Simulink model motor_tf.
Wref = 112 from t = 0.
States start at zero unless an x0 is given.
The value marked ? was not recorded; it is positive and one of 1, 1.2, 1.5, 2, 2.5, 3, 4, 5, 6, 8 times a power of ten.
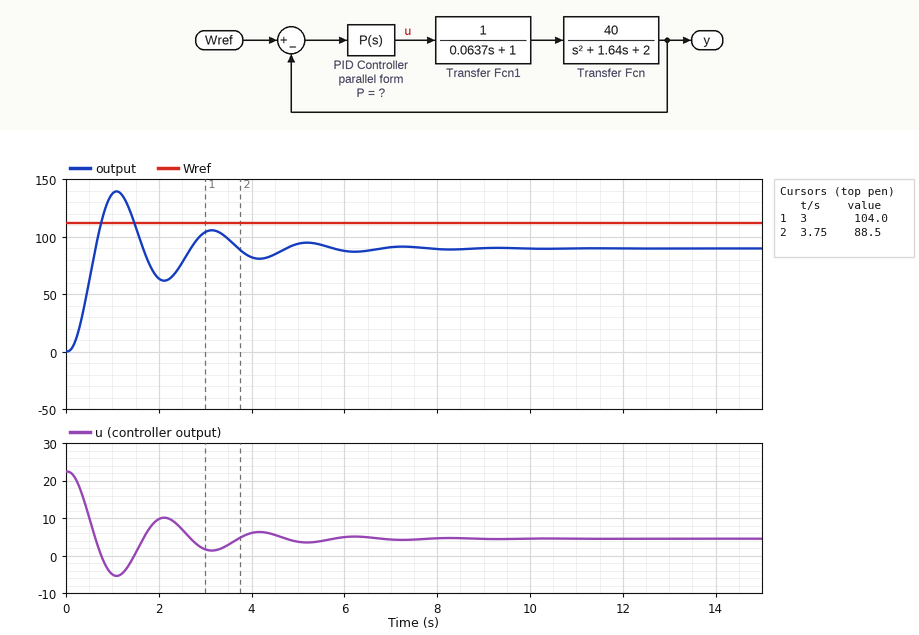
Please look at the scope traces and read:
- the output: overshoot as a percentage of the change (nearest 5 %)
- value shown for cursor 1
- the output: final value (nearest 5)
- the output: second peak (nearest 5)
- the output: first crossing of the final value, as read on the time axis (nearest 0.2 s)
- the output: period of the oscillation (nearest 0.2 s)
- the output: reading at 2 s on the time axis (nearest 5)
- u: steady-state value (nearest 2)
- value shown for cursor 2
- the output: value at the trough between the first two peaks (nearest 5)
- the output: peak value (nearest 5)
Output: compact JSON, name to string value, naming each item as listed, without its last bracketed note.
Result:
{"the output: overshoot as a percentage of the change": "55 %", "value shown for cursor 1": "104.0", "the output: final value": "90", "the output: second peak": "105", "the output: first crossing of the final value, as read on the time axis": "0.6 s", "the output: period of the oscillation": "2.0 s", "the output: reading at 2 s on the time axis": "65", "u: steady-state value": "4", "value shown for cursor 2": "88.5", "the output: value at the trough between the first two peaks": "60", "the output: peak value": "140"}
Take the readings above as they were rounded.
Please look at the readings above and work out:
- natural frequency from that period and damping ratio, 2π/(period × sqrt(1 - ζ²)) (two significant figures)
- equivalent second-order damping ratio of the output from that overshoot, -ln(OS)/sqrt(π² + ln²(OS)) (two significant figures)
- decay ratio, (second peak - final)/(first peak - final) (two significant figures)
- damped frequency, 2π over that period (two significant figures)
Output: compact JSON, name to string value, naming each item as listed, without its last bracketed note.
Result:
{"natural frequency from that period and damping ratio, 2π/(period × sqrt(1 - ζ²))": "3.2 rad/s", "equivalent second-order damping ratio of the output from that overshoot, -ln(OS)/sqrt(π² + ln²(OS))": "0.19", "decay ratio, (second peak - final)/(first peak - final)": "0.30", "damped frequency, 2π over that period": "3.1 rad/s"}
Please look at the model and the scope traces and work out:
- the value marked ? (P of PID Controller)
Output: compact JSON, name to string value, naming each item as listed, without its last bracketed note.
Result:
{"the value marked ?": "0.2"}
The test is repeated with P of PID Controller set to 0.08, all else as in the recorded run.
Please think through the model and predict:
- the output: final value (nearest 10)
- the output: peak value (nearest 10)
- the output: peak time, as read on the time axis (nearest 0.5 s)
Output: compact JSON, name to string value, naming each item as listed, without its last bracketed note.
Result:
{"the output: final value": "70", "the output: peak value": "90", "the output: peak time, as read on the time axis": "1.5 s"}
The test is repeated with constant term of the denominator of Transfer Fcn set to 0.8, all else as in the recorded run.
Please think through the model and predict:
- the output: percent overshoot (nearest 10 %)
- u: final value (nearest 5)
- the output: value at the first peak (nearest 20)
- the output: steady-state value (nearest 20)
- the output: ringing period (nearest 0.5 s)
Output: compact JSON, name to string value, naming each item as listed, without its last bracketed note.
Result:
{"the output: percent overshoot": "50 %", "u: final value": "0", "the output: value at the first peak": "160", "the output: steady-state value": "100", "the output: ringing period": "2.0 s"}
